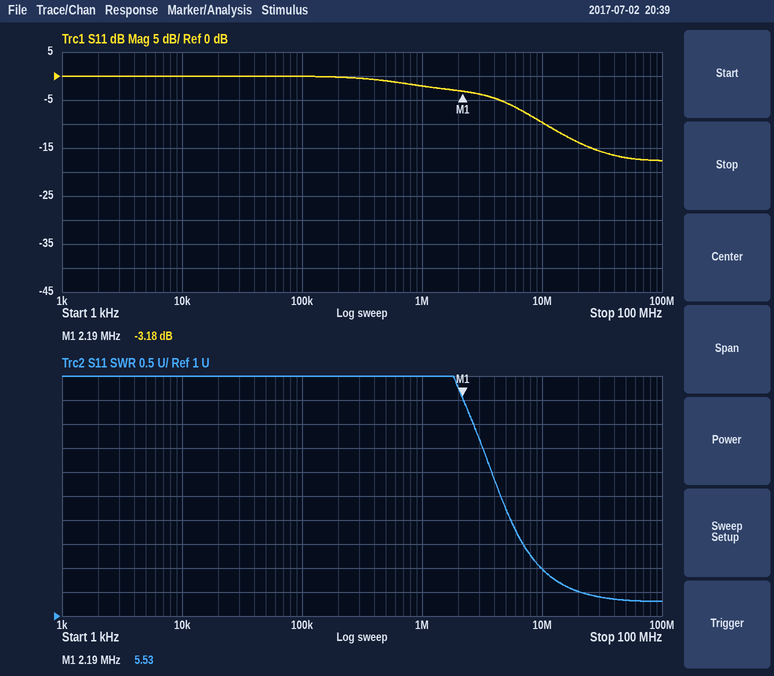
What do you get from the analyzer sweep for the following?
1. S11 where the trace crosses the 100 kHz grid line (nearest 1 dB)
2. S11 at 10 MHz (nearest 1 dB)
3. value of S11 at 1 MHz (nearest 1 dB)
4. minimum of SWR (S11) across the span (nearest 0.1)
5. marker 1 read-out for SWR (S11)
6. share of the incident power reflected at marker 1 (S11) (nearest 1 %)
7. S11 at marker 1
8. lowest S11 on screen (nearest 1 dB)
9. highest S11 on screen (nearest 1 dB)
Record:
0 dB
-10 dB
-2 dB
1.3
5.53
48 %
-3.18 dB
-18 dB
0 dB
